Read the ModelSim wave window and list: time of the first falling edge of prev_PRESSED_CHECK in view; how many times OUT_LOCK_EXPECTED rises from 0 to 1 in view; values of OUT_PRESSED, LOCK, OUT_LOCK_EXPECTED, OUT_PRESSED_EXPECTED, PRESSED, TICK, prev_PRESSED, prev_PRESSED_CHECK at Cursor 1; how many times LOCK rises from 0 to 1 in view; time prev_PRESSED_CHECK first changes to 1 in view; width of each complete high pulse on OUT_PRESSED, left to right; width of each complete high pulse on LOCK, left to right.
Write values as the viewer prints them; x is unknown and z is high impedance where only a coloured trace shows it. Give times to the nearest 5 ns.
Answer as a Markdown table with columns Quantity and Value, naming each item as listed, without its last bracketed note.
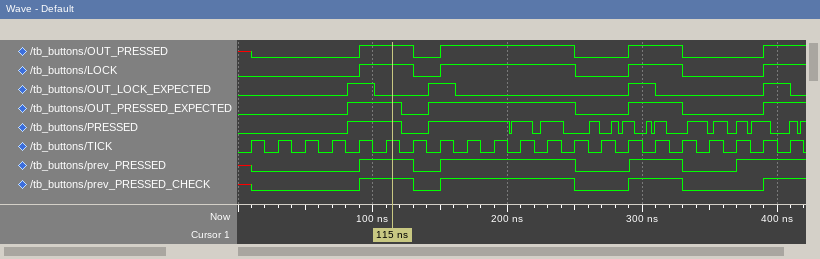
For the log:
| Quantity | Value |
|---|---|
| time of the first falling edge of prev_PRESSED_CHECK in view | 130 ns |
| how many times OUT_LOCK_EXPECTED rises from 0 to 1 in view | 4 |
| values of OUT_PRESSED, LOCK, OUT_LOCK_EXPECTED, OUT_PRESSED_EXPECTED, PRESSED, TICK, prev_PRESSED, prev_PRESSED_CHECK at Cursor 1 | OUT_PRESSED=1, LOCK=1, OUT_LOCK_EXPECTED=0, OUT_PRESSED_EXPECTED=1, PRESSED=1, TICK=1, prev_PRESSED=1, prev_PRESSED_CHECK=1 |
| how many times LOCK rises from 0 to 1 in view | 4 |
| time prev_PRESSED_CHECK first changes to 1 in view | 90 ns |
| width of each complete high pulse on OUT_PRESSED, left to right | 40 ns, 100 ns, 40 ns |
| width of each complete high pulse on LOCK, left to right | 40 ns, 100 ns, 40 ns |
